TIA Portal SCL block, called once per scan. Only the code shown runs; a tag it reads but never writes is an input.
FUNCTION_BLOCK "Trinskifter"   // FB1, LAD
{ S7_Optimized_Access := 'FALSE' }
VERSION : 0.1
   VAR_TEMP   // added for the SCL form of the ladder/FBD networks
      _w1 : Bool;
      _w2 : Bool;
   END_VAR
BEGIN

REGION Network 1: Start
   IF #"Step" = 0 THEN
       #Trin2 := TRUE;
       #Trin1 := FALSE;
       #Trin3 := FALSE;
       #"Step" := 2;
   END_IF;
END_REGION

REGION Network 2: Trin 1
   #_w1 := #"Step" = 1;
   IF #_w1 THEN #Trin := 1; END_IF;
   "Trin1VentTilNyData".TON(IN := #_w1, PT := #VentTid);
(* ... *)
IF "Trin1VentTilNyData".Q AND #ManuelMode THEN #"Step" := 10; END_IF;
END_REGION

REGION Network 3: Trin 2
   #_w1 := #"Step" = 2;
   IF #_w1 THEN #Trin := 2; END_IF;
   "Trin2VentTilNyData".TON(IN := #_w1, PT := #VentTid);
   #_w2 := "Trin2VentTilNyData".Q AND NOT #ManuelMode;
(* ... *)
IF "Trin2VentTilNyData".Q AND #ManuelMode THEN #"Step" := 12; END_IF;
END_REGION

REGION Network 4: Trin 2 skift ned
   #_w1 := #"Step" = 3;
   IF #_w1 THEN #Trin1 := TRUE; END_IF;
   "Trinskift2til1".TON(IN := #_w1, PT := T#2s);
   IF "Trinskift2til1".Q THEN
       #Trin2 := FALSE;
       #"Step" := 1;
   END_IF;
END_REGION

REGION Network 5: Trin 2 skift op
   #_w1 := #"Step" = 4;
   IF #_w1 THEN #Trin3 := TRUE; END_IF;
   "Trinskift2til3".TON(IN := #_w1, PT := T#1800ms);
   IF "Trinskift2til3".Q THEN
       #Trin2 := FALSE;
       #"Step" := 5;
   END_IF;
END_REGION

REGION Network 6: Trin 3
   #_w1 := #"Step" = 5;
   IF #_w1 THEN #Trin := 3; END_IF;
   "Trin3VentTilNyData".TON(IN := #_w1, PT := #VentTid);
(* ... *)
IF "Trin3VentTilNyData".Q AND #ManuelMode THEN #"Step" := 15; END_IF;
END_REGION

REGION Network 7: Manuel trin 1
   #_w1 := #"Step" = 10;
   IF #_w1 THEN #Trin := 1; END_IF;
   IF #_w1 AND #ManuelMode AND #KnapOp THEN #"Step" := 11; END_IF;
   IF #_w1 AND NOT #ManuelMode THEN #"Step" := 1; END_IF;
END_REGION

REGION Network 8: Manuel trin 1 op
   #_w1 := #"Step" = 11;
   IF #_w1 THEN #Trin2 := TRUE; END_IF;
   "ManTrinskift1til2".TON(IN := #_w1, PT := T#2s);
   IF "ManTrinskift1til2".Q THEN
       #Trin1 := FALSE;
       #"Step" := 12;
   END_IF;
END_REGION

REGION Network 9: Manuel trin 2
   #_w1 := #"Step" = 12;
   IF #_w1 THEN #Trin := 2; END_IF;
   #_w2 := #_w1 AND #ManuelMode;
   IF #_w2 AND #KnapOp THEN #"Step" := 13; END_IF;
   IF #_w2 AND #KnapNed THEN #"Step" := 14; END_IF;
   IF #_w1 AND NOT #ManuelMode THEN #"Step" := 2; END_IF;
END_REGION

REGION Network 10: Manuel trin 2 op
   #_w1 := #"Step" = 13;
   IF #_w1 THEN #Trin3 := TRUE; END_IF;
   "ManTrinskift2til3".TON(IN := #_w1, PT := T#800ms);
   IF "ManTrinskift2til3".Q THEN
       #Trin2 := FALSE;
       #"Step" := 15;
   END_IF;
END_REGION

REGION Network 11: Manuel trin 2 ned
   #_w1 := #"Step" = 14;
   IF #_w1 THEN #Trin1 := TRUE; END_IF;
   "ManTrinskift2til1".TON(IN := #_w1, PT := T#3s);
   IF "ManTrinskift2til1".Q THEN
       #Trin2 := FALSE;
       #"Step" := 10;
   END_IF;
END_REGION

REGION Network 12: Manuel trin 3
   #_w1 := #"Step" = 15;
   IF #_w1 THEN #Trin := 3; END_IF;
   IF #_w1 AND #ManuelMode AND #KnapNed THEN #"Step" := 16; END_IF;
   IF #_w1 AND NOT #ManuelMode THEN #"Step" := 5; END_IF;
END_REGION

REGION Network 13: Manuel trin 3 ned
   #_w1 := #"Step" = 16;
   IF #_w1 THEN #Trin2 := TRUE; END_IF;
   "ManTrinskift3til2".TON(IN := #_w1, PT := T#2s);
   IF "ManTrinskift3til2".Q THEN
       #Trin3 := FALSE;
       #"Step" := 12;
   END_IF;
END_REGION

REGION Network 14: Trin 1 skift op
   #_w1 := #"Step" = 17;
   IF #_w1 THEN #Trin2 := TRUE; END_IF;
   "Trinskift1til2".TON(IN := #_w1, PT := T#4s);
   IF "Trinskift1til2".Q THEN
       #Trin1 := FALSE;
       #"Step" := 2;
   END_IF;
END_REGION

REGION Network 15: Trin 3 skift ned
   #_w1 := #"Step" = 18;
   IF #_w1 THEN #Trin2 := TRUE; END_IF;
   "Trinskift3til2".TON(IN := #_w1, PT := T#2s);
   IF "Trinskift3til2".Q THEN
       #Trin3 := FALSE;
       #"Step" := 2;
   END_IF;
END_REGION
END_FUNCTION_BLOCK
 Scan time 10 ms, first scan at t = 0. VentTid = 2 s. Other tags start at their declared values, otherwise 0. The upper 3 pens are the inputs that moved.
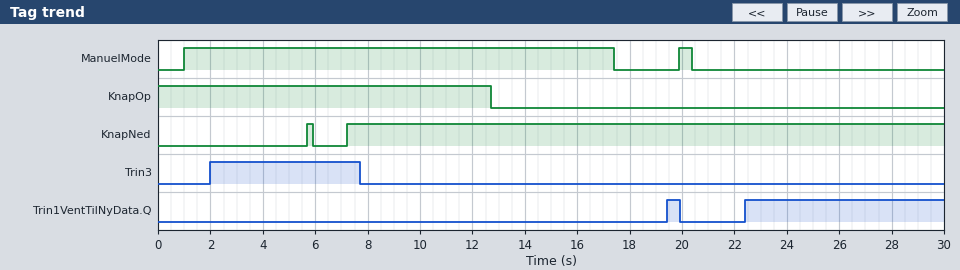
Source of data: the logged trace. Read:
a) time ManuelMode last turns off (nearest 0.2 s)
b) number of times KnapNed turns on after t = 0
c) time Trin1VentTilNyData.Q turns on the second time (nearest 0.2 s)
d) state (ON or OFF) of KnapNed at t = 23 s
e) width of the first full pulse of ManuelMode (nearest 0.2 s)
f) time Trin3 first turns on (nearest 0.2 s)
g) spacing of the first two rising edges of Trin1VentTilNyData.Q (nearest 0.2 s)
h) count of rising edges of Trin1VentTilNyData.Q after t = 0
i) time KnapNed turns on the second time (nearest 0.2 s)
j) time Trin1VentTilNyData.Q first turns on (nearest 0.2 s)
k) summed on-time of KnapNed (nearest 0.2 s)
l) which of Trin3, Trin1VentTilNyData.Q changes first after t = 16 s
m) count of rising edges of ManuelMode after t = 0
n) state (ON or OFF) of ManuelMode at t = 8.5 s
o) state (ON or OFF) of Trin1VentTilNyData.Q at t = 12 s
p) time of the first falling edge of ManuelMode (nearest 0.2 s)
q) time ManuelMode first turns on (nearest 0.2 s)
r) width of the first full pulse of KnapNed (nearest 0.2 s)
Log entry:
20.4 s
2
22.4 s
ON
16.4 s
2.0 s
3.0 s
2
7.2 s
19.4 s
23.0 s
Trin1VentTilNyData.Q
2
ON
OFF
17.4 s
1.0 s
0.2 s
